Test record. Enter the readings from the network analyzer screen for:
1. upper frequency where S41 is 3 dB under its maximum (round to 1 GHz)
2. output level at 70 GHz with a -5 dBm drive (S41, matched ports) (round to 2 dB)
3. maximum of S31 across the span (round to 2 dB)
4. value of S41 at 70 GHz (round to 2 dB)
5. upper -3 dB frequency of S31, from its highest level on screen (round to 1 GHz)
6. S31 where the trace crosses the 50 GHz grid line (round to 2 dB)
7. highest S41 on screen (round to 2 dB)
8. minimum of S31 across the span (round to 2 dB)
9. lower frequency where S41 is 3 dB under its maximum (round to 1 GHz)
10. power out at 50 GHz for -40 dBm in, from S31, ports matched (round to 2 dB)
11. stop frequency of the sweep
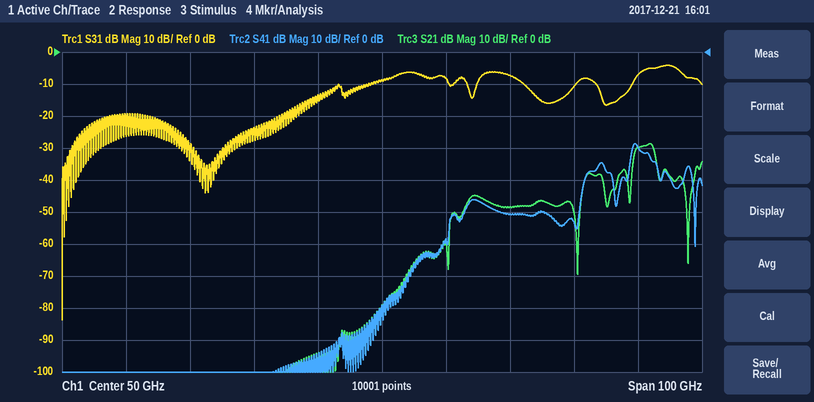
91 GHz
-56 dBm
-4 dB
-50 dB
97 GHz
-8 dB
-28 dB
-84 dB
89 GHz
-48 dBm
100 GHz
